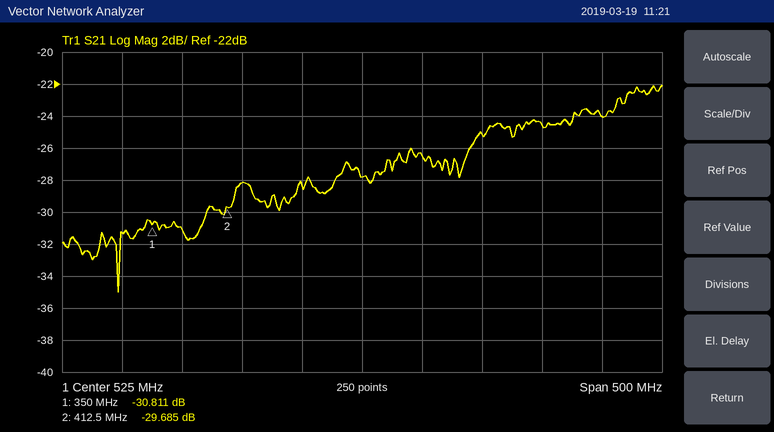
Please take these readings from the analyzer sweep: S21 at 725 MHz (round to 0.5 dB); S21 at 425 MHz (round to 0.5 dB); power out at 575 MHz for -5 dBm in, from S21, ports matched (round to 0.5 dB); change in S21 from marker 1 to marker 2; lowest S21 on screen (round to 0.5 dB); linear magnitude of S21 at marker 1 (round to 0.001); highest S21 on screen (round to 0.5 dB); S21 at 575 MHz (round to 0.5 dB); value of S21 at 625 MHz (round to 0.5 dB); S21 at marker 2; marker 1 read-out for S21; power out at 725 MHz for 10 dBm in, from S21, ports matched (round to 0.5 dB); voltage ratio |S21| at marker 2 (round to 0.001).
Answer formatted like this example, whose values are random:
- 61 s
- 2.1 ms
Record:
- -24.0 dB
- -28.0 dB
- -31.5 dBm
- 1.126 dB
- -35.0 dB
- 0.029
- -22.0 dB
- -26.5 dB
- -25.0 dB
- -29.685 dB
- -30.811 dB
- -14.0 dBm
- 0.033
